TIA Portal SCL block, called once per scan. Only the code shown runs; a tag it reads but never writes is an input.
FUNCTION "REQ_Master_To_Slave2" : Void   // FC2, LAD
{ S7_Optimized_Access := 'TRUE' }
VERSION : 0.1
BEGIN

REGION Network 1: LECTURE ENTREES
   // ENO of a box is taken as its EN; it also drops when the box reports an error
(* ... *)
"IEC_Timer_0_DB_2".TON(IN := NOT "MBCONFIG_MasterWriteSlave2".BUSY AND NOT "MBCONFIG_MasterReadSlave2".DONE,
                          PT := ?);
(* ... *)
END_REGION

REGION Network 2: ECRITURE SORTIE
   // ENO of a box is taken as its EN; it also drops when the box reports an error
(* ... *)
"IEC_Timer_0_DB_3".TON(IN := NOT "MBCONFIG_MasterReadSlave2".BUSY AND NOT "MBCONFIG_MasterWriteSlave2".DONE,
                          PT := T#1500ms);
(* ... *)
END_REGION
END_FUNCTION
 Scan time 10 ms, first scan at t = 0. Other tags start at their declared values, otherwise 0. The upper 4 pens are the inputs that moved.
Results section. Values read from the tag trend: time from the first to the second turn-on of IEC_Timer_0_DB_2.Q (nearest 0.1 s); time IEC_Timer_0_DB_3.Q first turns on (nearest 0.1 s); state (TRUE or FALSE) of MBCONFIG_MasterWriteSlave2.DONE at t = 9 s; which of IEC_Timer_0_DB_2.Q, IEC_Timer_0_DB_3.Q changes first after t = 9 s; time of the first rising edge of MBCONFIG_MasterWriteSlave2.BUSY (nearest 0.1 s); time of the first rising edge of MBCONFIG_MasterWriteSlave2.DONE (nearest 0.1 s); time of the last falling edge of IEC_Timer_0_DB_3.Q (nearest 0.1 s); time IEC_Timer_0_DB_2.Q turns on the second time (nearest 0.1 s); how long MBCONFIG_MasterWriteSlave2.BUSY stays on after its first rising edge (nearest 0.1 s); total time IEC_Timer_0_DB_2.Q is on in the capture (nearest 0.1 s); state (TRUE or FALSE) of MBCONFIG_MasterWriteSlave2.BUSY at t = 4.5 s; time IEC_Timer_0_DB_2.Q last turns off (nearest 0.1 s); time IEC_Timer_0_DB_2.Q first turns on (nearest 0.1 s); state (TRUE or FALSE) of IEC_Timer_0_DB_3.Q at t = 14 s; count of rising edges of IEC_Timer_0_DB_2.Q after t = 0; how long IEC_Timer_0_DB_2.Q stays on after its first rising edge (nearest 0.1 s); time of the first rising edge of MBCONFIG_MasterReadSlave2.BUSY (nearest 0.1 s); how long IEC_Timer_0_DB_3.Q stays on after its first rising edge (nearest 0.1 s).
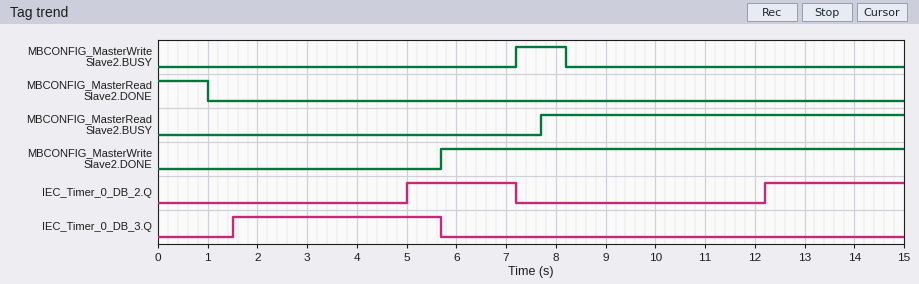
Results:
7.2 s
1.5 s
TRUE
IEC_Timer_0_DB_2.Q
7.2 s
5.7 s
5.7 s
12.2 s
1.0 s
5.0 s
FALSE
7.2 s
5.0 s
FALSE
2
2.2 s
7.7 s
4.2 s
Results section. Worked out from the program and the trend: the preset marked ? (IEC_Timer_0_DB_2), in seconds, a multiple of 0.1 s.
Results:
4.0 s
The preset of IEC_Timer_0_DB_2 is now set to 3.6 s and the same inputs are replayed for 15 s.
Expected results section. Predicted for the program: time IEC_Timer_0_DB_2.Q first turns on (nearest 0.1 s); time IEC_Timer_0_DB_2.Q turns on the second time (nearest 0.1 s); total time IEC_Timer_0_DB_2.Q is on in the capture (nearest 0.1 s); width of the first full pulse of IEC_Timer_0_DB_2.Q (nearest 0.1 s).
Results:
4.6 s
11.8 s
5.8 s
2.6 s
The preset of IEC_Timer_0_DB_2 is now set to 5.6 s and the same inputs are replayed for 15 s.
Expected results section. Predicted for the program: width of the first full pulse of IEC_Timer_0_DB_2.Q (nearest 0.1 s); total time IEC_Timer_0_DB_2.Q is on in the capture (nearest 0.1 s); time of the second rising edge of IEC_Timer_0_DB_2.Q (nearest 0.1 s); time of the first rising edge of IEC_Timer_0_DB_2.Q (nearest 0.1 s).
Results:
0.6 s
1.8 s
13.8 s
6.6 s
